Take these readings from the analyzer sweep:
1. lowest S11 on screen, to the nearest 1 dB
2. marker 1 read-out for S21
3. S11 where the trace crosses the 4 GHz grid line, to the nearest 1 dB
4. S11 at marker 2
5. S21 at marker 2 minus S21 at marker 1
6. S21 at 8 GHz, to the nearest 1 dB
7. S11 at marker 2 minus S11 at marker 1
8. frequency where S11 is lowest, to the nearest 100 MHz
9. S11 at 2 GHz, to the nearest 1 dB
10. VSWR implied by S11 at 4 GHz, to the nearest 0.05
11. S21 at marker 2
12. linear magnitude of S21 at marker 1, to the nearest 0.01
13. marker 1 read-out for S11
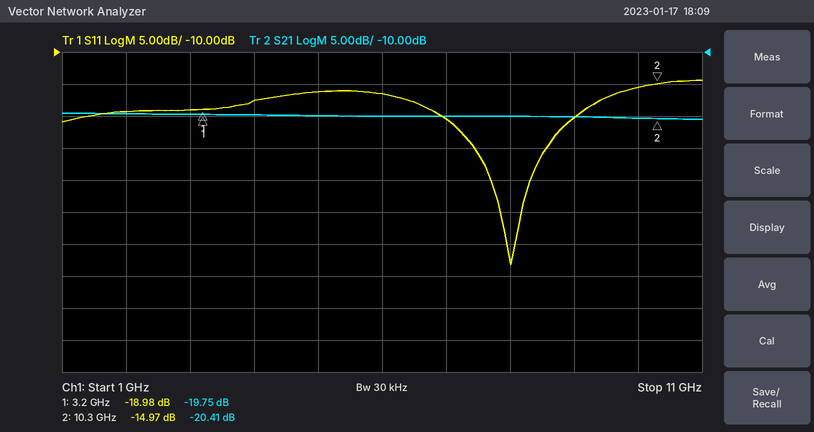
-43 dB
-19.75 dB
-18 dB
-14.97 dB
-0.66 dB
-20 dB
4.01 dB
8.0 GHz
-19 dB
1.30
-20.41 dB
0.10
-18.98 dB
